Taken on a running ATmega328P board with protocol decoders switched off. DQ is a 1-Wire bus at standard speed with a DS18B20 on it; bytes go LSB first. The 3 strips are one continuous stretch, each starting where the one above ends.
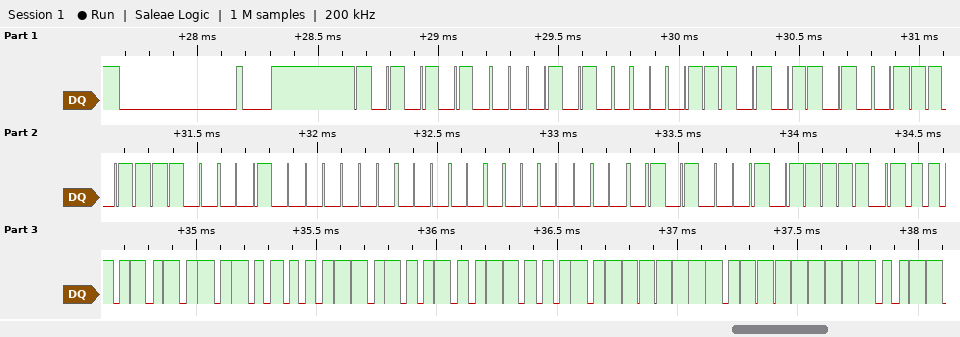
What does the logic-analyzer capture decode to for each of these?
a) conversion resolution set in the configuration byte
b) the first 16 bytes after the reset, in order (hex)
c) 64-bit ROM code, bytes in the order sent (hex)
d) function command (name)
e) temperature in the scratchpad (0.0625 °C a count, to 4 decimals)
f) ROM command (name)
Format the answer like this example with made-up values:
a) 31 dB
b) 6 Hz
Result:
a) 12 bits
b) 55 28 B8 96 7B 08 00 00 8A BE 50 05 4B 46 7F FF
c) 28 B8 96 7B 08 00 00 8A
d) Read Scratchpad
e) 85.0000 °C
f) Match ROM
